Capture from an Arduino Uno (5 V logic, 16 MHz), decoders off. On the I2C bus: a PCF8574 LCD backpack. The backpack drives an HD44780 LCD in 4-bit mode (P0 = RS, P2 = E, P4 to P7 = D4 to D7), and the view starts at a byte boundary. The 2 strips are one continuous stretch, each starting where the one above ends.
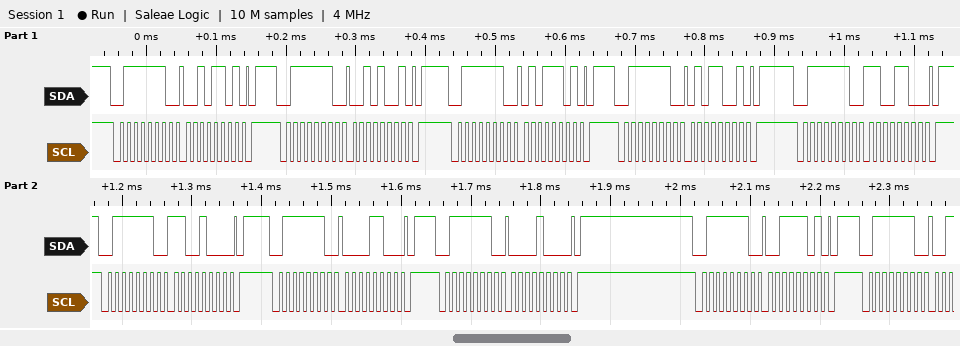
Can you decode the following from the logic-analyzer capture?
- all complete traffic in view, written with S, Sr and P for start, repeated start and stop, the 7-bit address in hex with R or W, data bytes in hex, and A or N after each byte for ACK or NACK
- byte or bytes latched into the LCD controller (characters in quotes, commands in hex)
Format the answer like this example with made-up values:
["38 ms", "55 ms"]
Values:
["S 3FW A 2D A P S 3FW A 29 A P S 3FW A 5D A P S 3FW A 59 A P S 3FW A CC A P S 3FW A C8 A P S 3FW A 0C A P S 3FW A 08 A P S 3FW A 3D A P S 3FW A", "'%' 0xC0"]
